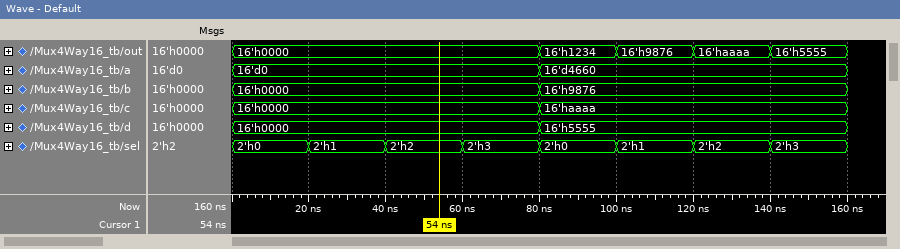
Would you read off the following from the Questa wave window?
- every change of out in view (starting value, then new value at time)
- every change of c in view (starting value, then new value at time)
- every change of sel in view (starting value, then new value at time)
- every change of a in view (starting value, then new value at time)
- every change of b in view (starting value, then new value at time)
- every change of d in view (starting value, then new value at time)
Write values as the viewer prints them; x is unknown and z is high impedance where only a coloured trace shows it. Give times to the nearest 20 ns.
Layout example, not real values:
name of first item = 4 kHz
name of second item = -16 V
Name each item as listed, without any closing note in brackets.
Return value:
every change of out in view = 16'h0000, 16'h1234 at 80 ns, 16'h9876 at 100 ns, 16'haaaa at 120 ns, 16'h5555 at 140 ns
every change of c in view = 16'h0000, 16'haaaa at 80 ns
every change of sel in view = 2'h0, 2'h1 at 20 ns, 2'h2 at 40 ns, 2'h3 at 60 ns, 2'h0 at 80 ns, 2'h1 at 100 ns, 2'h2 at 120 ns, 2'h3 at 140 ns
every change of a in view = 16'd0, 16'd4660 at 80 ns
every change of b in view = 16'h0000, 16'h9876 at 80 ns
every change of d in view = 16'h0000, 16'h5555 at 80 ns
